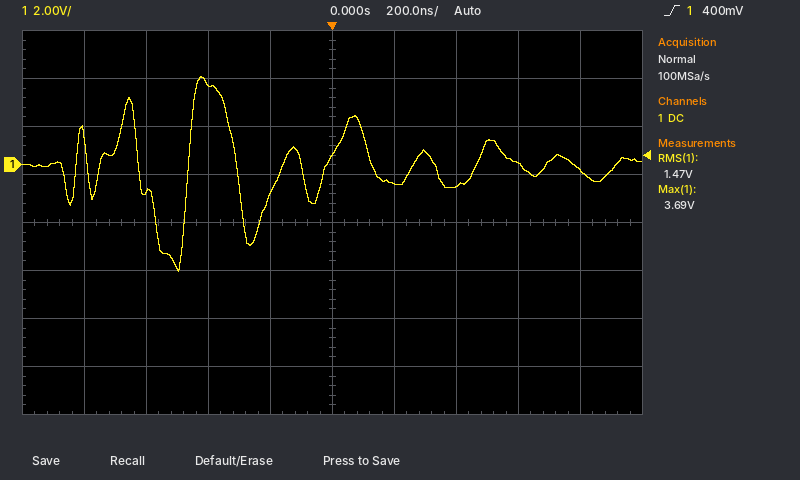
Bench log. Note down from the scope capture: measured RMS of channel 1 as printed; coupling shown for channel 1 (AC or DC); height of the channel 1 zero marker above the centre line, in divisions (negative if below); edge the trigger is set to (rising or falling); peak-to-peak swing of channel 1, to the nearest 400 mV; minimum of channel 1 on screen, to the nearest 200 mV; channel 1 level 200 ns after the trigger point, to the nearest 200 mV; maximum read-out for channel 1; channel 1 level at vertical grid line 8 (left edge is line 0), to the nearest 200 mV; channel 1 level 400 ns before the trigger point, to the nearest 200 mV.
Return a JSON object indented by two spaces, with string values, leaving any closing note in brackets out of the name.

{
  "measured RMS of channel 1 as printed": "1.47 V",
  "coupling shown for channel 1": "DC",
  "height of the channel 1 zero marker above the centre line, in divisions": "+1.2 div",
  "edge the trigger is set to": "rising",
  "peak-to-peak swing of channel 1, to the nearest 400 mV": "8.0 V",
  "minimum of channel 1 on screen, to the nearest 200 mV": "-4.4 V",
  "channel 1 level 200 ns after the trigger point, to the nearest 200 mV": "-800 mV",
  "maximum read-out for channel 1": "3.69 V",
  "channel 1 level at vertical grid line 8 (left edge is line 0), to the nearest 200 mV": "0.0 V",
  "channel 1 level 400 ns before the trigger point, to the nearest 200 mV": "3.4 V"
}
